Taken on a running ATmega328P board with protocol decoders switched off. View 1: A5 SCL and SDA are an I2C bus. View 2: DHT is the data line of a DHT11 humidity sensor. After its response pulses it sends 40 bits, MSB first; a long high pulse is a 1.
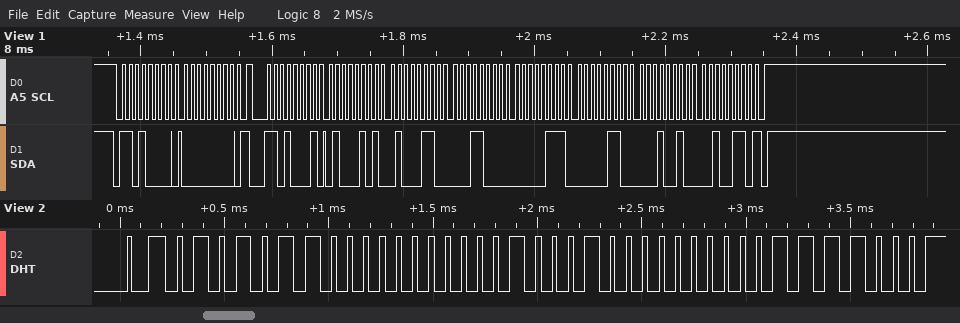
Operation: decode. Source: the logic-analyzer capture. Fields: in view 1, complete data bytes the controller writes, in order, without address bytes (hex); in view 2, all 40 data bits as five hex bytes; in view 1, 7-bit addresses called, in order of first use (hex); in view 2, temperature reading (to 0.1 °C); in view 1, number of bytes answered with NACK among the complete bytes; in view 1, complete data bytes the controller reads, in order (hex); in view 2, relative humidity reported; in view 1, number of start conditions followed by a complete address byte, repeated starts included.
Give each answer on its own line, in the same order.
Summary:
00
56 00 22 00 78
0x68
34.0 °C
1
45 46 18 07 06 12 26
86 %
2
